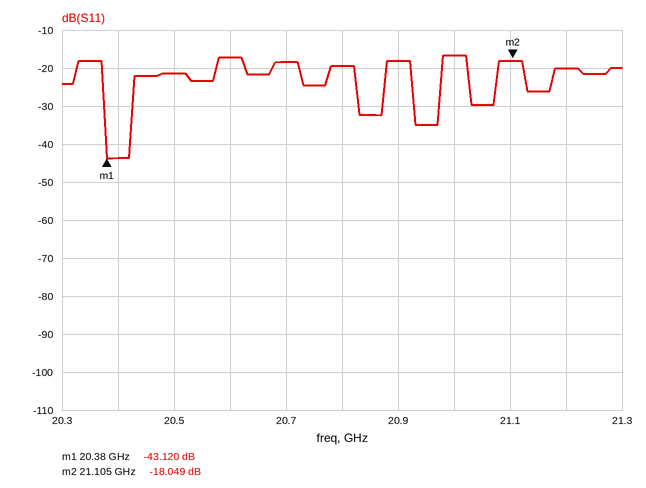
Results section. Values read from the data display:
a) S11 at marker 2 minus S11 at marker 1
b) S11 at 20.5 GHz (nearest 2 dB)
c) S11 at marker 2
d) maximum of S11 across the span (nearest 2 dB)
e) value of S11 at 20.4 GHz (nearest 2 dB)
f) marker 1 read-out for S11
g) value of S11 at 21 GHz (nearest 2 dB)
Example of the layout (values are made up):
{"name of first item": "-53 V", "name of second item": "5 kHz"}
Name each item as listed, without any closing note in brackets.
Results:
{"S11 at marker 2 minus S11 at marker 1": "25.071 dB", "S11 at 20.5 GHz": "-22 dB", "S11 at marker 2": "-18.049 dB", "maximum of S11 across the span": "-16 dB", "value of S11 at 20.4 GHz": "-44 dB", "marker 1 read-out for S11": "-43.120 dB", "value of S11 at 21 GHz": "-16 dB"}
